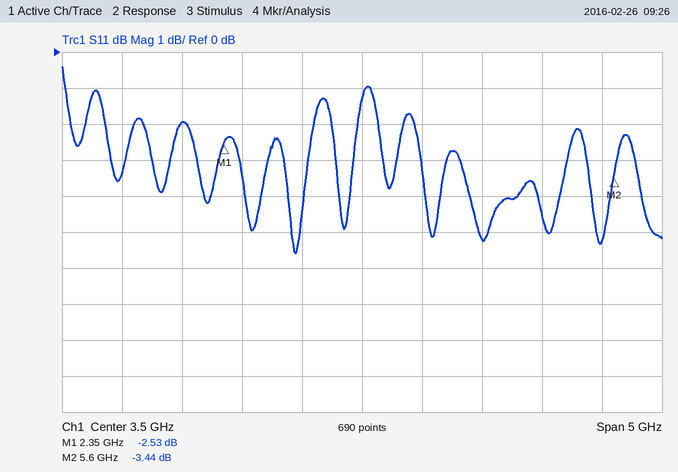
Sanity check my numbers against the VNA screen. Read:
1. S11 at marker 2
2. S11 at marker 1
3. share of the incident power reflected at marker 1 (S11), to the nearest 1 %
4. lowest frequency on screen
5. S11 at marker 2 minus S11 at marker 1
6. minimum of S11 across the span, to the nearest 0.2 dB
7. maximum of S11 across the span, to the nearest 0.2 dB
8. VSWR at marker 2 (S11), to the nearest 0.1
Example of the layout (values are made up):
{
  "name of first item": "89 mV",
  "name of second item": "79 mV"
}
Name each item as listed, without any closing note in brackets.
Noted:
{
  "S11 at marker 2": "-3.44 dB",
  "S11 at marker 1": "-2.53 dB",
  "share of the incident power reflected at marker 1 (S11), to the nearest 1 %": "56 %",
  "lowest frequency on screen": "1 GHz",
  "S11 at marker 2 minus S11 at marker 1": "-0.91 dB",
  "minimum of S11 across the span, to the nearest 0.2 dB": "-5.6 dB",
  "maximum of S11 across the span, to the nearest 0.2 dB": "-0.4 dB",
  "VSWR at marker 2 (S11), to the nearest 0.1": "5.1"
}
